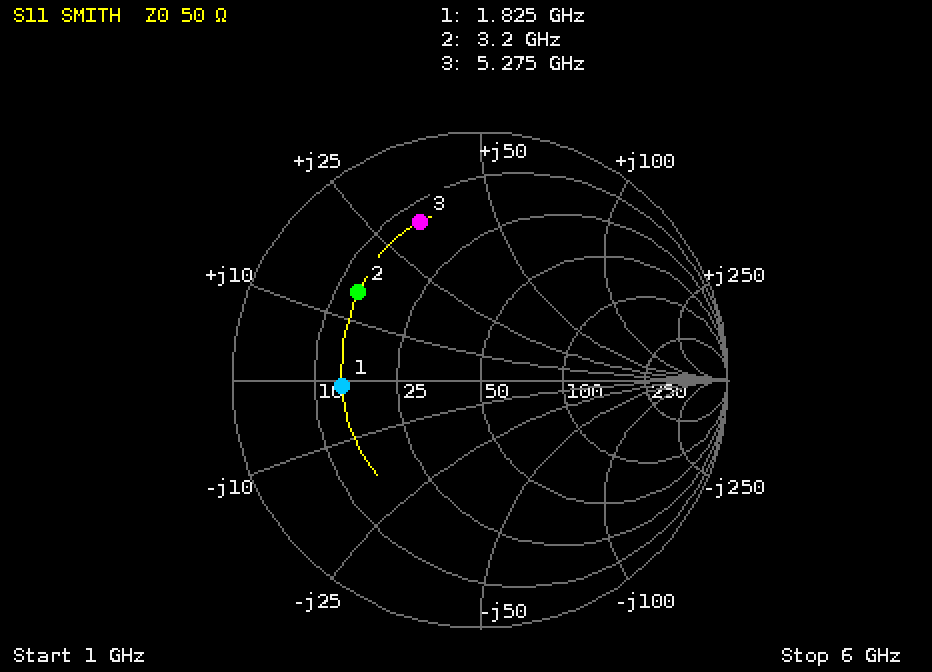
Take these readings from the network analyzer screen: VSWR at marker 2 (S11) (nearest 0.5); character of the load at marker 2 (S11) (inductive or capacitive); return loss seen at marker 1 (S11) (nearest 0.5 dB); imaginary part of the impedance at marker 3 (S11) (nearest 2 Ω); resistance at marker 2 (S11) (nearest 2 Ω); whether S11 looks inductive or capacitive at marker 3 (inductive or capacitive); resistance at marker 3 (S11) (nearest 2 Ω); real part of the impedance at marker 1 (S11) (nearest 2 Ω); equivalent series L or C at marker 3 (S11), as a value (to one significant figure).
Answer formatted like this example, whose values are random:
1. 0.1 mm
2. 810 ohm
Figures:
1. 4.0
2. inductive
3. 5.0 dB
4. +32 Ω
5. 14 Ω
6. inductive
7. 14 Ω
8. 14 Ω
9. 1.0 nH
